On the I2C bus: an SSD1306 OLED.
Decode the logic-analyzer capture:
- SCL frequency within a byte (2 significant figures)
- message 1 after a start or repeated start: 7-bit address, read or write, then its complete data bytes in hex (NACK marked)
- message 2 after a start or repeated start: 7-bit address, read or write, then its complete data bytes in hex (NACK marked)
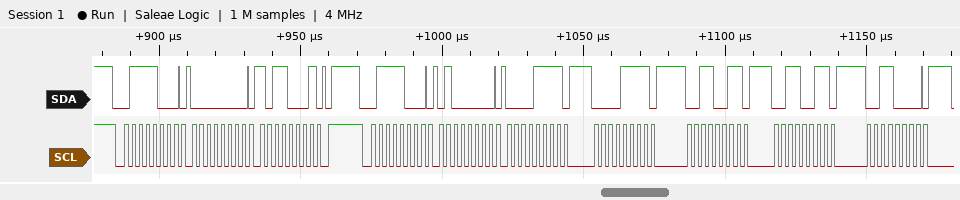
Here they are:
400 kHz
0x3C write: 00 B1
0x3C write: 40 0F 0F 33 33 30
